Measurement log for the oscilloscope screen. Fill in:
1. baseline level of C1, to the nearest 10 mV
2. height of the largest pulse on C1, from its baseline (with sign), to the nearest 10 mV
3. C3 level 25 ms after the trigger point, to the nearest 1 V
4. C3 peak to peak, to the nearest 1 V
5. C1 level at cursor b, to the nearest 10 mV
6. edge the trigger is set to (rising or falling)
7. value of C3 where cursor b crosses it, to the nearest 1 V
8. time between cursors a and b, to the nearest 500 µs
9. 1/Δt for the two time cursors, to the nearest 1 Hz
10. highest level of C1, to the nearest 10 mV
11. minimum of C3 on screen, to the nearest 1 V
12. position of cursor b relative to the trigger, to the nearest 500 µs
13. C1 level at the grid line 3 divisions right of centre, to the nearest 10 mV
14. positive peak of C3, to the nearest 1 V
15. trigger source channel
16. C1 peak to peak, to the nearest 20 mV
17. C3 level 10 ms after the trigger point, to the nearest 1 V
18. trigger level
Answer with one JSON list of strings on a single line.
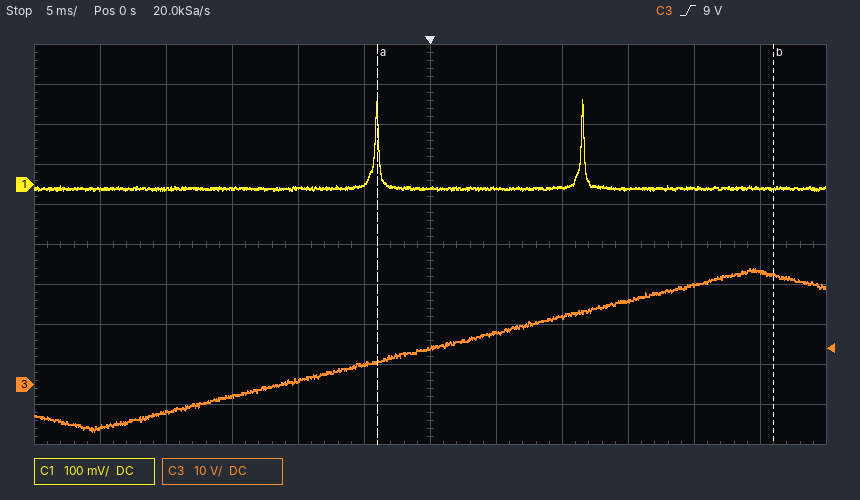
["-10 mV", "+220 mV", "28 V", "41 V", "-10 mV", "rising", "27 V", "30.0 ms", "33 Hz", "210 mV", "-12 V", "+26.0 ms", "-10 mV", "29 V", "C3", "220 mV", "17 V", "9 V"]
